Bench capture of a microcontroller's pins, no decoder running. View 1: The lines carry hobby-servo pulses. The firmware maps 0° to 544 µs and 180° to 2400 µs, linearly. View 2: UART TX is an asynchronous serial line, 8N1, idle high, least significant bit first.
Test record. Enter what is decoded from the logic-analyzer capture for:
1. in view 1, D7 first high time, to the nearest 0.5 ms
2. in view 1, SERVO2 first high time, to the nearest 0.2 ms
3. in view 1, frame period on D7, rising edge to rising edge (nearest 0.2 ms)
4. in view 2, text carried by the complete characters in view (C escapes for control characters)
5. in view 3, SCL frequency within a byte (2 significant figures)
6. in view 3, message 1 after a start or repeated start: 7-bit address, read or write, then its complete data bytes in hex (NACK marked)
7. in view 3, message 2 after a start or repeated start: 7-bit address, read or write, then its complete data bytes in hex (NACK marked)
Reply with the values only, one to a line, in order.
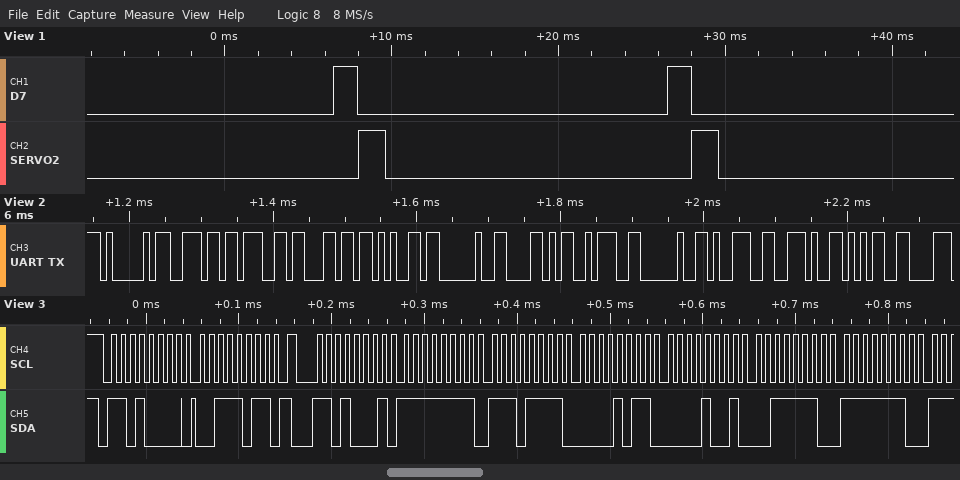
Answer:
1.5 ms
1.6 ms
20.0 ms
"Angle X: 9.5"
100 kHz
0x68 write: 3B
0x68 read: FF EF 0B 09 3E FE
